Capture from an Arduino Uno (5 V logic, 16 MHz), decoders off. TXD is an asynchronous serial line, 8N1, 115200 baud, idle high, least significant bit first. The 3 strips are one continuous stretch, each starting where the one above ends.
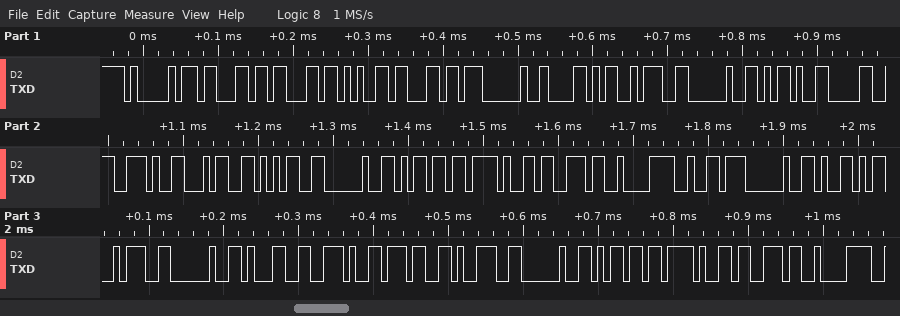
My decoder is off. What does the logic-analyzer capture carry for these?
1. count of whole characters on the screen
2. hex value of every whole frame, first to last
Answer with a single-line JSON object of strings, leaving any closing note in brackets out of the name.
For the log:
{"count of whole characters on the screen": "33", "hex value of every whole frame, first to last": "0x41 0x63 0x63 0x65 0x6C 0x20 0x58 0x3A 0x20 0x2D 0x30 0x2E 0x34 0x35 0x20 0x6D 0x2F 0x73 0xC2 0xB2 0x20 0x59 0x3A 0x20 0x31 0x2E 0x37 0x39 0x20 0x6D 0x2F 0x73 0xC2"}
